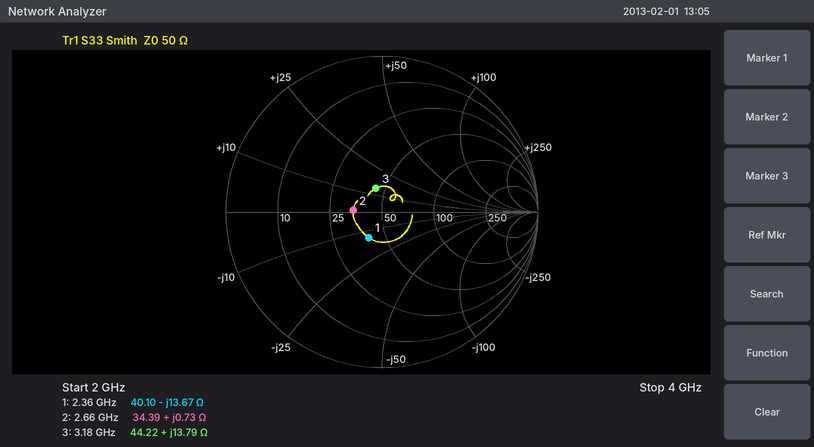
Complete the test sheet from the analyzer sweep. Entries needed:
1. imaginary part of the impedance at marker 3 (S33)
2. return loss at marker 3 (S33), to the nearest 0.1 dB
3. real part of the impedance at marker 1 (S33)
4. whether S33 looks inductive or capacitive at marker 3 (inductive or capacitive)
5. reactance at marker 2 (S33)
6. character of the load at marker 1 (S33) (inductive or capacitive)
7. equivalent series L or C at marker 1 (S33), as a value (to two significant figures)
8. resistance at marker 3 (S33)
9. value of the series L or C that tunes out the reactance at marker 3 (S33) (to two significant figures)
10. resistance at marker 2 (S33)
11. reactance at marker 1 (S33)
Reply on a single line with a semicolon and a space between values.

+13.79 Ω; 16.1 dB; 40.10 Ω; inductive; +0.73 Ω; capacitive; 4.9 pF; 44.22 Ω; 3.6 pF; 34.39 Ω; -13.67 Ω
